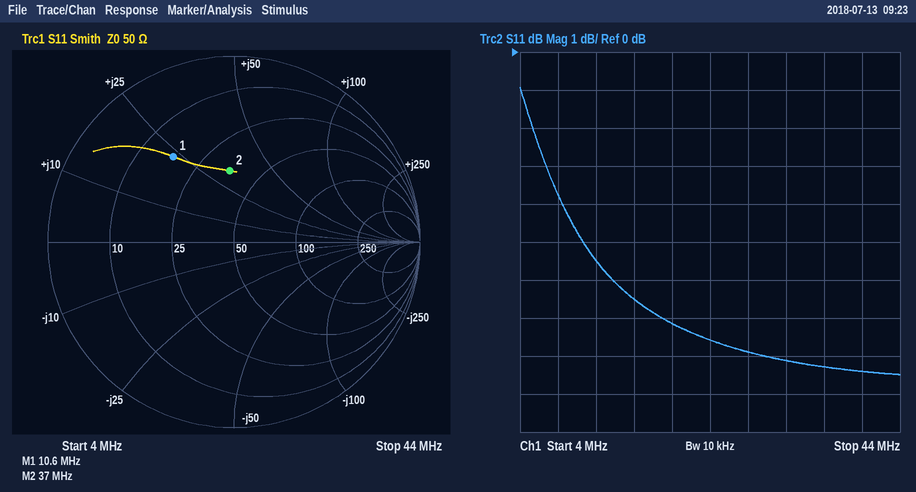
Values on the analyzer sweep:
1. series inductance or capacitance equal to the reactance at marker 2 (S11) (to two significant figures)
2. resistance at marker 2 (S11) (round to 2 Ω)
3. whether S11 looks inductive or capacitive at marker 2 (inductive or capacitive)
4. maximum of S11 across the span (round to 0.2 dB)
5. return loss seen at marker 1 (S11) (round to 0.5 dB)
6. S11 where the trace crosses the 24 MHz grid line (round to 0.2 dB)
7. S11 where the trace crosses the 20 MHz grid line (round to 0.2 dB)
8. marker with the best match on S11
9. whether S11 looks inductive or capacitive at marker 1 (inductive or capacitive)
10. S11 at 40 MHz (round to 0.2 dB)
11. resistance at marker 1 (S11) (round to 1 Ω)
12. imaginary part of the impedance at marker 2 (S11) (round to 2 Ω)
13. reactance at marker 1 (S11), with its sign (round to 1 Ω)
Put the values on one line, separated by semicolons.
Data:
140 nH; 36 Ω; inductive; -1.0 dB; 5.0 dB; -7.6 dB; -7.2 dB; marker 2; inductive; -8.4 dB; 17 Ω; +32 Ω; +23 Ω
